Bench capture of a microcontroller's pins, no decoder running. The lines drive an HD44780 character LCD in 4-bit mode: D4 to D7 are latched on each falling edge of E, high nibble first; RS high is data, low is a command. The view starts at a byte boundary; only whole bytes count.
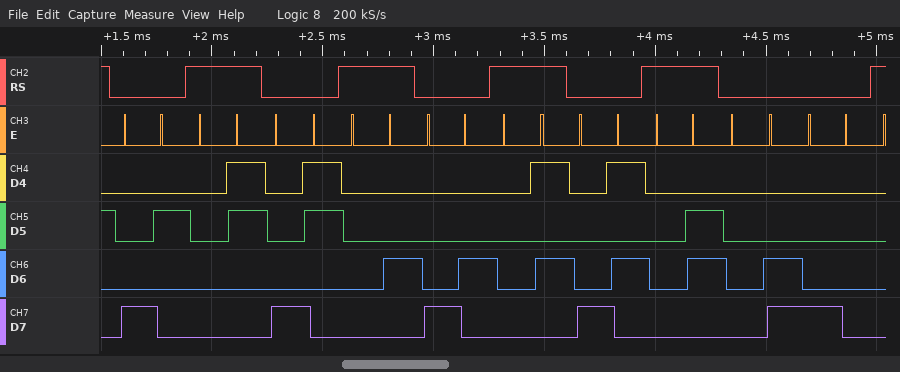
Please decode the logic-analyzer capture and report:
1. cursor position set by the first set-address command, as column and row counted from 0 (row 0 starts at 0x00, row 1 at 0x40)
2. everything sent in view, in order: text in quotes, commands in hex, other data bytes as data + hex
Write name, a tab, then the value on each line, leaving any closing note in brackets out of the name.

cursor position set by the first set-address command, as column and row counted from 0	column 2, row 0
everything sent in view, in order: text in quotes, commands in hex, other data bytes as data + hex	0x82 data 03 0x83 data 04 0x84 data 05 0x85 data 06 0x0C 0x80
